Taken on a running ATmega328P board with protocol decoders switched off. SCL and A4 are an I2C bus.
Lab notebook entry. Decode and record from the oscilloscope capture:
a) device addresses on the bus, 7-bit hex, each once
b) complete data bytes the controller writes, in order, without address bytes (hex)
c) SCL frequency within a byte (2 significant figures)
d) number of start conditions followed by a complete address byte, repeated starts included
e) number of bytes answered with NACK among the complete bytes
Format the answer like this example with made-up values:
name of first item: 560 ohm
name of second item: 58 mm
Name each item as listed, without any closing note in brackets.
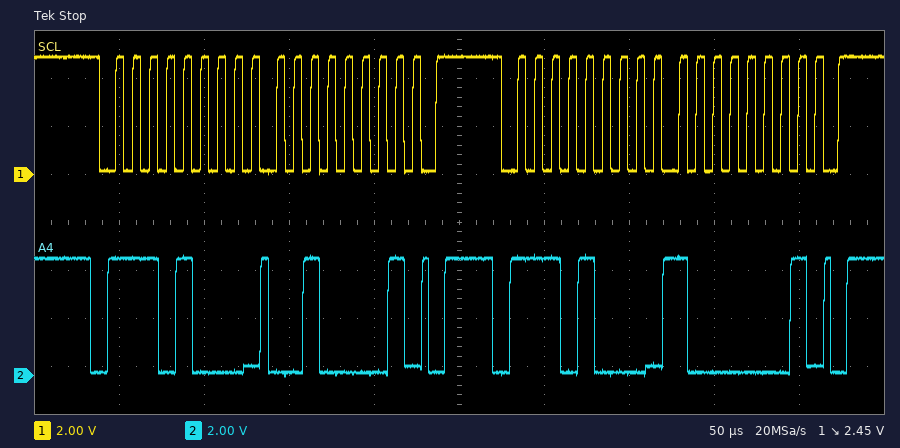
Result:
device addresses on the bus, 7-bit hex, each once: 0x74
complete data bytes the controller writes, in order, without address bytes: 21 81
SCL frequency within a byte: 100 kHz
number of start conditions followed by a complete address byte, repeated starts included: 2
number of bytes answered with NACK among the complete bytes: 0
